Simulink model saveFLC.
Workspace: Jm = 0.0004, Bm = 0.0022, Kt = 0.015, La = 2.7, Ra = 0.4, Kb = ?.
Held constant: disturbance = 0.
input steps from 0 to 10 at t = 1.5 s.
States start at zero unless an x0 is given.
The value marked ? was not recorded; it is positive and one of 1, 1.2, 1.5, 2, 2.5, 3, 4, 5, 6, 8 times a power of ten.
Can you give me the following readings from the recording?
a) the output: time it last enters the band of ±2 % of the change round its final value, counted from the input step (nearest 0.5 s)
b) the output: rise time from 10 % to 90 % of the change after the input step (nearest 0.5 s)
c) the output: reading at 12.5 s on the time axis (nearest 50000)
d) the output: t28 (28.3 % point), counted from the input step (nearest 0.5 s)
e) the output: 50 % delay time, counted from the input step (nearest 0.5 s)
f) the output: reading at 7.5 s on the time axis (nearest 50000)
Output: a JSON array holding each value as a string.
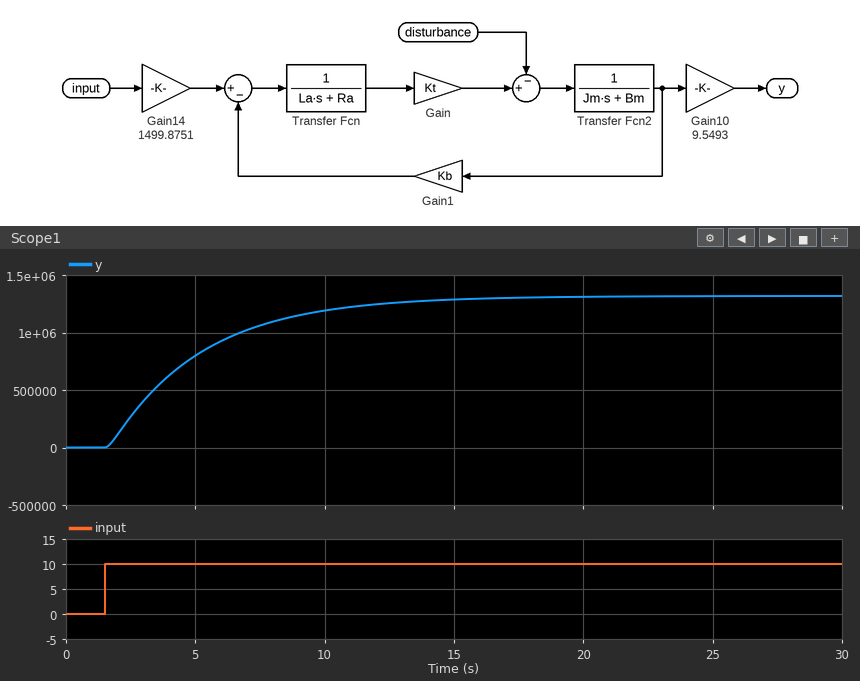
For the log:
["14.0 s", "8.0 s", "1250000", "1.5 s", "2.5 s", "1050000"]
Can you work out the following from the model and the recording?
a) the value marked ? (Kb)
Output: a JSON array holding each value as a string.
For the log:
["0.05"]
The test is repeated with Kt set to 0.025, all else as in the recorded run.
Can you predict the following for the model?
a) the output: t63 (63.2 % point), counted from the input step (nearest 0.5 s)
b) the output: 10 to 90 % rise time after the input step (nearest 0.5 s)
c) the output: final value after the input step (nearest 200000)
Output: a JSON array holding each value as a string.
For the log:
["3.0 s", "6.0 s", "1600000"]
